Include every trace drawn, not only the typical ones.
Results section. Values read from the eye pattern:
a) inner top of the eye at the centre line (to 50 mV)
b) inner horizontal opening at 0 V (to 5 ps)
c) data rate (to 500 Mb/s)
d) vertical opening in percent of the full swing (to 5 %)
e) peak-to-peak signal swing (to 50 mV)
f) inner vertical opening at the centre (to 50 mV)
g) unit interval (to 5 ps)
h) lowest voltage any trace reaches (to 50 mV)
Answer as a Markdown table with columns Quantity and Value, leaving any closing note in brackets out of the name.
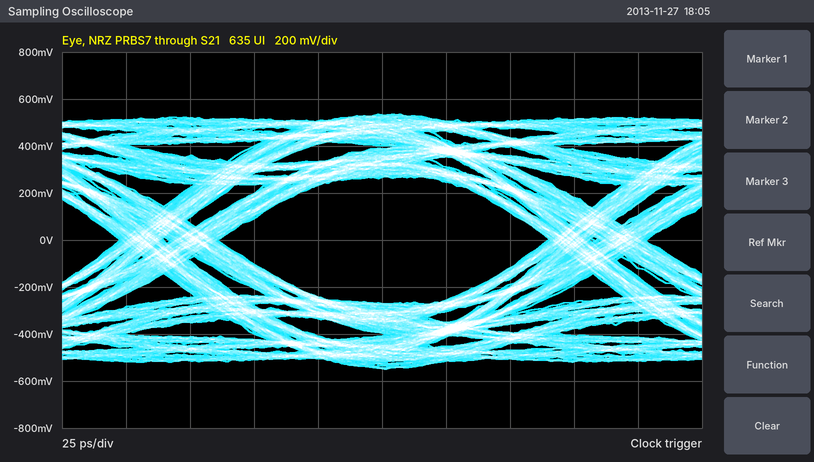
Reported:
| Quantity | Value |
|---|---|
| inner top of the eye at the centre line | 250 mV |
| inner horizontal opening at 0 V | 130 ps |
| data rate | 6.0 Gb/s |
| vertical opening in percent of the full swing | 50 % |
| peak-to-peak signal swing | 1.10 V |
| inner vertical opening at the centre | 550 mV |
| unit interval | 165 ps |
| lowest voltage any trace reaches | -550 mV |
